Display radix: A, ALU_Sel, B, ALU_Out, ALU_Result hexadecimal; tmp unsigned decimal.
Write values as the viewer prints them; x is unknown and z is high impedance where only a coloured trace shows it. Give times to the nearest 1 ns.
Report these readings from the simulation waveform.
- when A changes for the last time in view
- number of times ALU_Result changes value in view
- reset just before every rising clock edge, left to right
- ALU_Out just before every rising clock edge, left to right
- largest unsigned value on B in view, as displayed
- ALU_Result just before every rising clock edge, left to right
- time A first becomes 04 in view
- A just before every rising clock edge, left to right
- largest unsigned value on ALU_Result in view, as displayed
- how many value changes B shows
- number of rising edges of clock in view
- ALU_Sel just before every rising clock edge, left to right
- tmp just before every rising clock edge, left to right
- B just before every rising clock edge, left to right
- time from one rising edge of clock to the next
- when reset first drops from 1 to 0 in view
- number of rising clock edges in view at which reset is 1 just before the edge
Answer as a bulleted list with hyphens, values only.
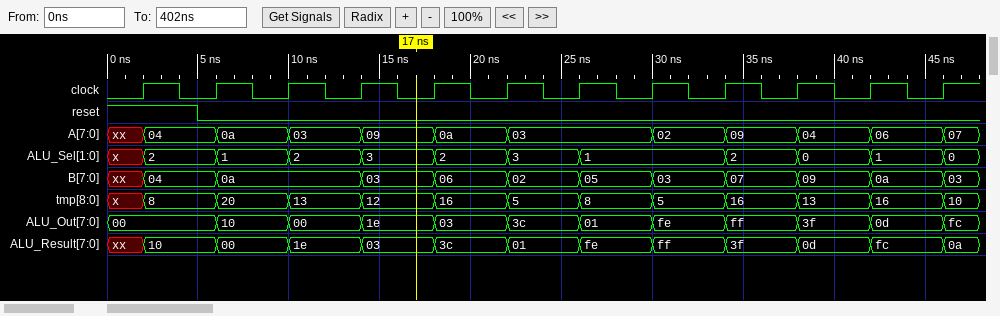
- 46 ns
- 12
- 1 0 0 0 0 0 0 0 0 0 0 0
- 00, 00, 10, 00, 1e, 03, 3c, 01, fe, ff, 3f, 0d
- 0a
- xx, 10, 00, 1e, 03, 3c, 01, fe, ff, 3f, 0d, fc
- 2 ns
- xx, 04, 0a, 03, 09, 0a, 03, 03, 02, 09, 04, 06
- ff
- 11
- 12
- x, 2, 1, 2, 3, 2, 3, 1, 1, 2, 0, 1
- x, 8, 20, 13, 12, 16, 5, 8, 5, 16, 13, 16
- xx, 04, 0a, 0a, 03, 06, 02, 05, 03, 07, 09, 0a
- 4 ns
- 5 ns
- 1
